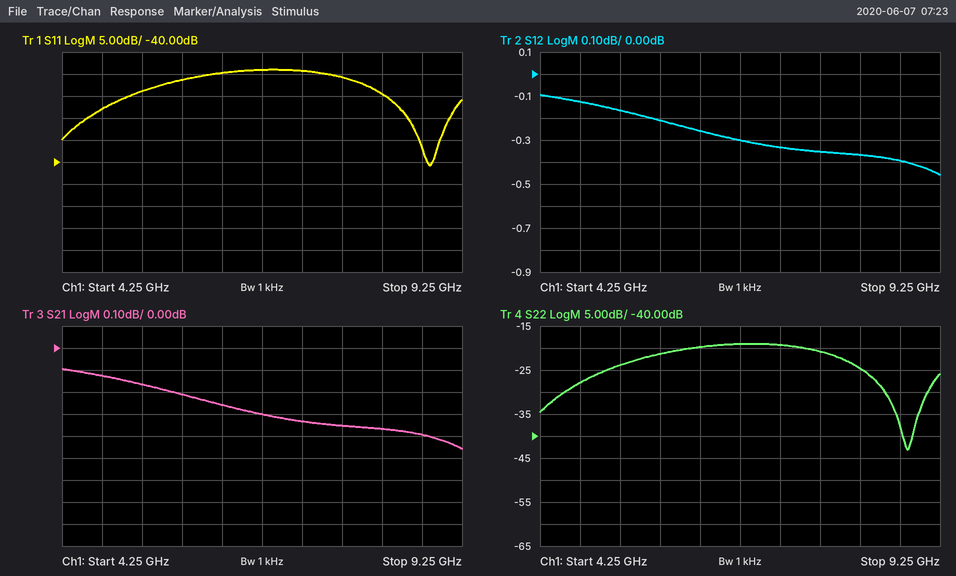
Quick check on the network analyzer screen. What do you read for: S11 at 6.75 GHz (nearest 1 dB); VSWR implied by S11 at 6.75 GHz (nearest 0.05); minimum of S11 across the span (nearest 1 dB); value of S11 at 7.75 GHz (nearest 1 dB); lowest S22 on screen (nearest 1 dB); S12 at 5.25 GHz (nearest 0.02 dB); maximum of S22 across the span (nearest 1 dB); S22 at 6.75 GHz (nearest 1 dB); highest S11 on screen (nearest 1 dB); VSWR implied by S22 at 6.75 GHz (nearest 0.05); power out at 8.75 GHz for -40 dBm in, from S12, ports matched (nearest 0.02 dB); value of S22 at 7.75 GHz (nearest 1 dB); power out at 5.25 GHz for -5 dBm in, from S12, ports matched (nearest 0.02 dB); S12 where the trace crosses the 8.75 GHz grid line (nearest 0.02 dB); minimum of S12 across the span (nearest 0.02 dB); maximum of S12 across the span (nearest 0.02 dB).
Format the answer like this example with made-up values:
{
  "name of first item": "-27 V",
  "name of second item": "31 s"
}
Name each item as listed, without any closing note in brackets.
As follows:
{
  "S11 at 6.75 GHz": "-19 dB",
  "VSWR implied by S11 at 6.75 GHz": "1.25",
  "minimum of S11 across the span": "-41 dB",
  "value of S11 at 7.75 GHz": "-21 dB",
  "lowest S22 on screen": "-43 dB",
  "S12 at 5.25 GHz": "-0.16 dB",
  "maximum of S22 across the span": "-19 dB",
  "S22 at 6.75 GHz": "-19 dB",
  "highest S11 on screen": "-19 dB",
  "VSWR implied by S22 at 6.75 GHz": "1.25",
  "power out at 8.75 GHz for -40 dBm in, from S12, ports matched": "-40.40 dBm",
  "value of S22 at 7.75 GHz": "-21 dB",
  "power out at 5.25 GHz for -5 dBm in, from S12, ports matched": "-5.16 dBm",
  "S12 where the trace crosses the 8.75 GHz grid line": "-0.40 dB",
  "minimum of S12 across the span": "-0.46 dB",
  "maximum of S12 across the span": "-0.10 dB"
}
